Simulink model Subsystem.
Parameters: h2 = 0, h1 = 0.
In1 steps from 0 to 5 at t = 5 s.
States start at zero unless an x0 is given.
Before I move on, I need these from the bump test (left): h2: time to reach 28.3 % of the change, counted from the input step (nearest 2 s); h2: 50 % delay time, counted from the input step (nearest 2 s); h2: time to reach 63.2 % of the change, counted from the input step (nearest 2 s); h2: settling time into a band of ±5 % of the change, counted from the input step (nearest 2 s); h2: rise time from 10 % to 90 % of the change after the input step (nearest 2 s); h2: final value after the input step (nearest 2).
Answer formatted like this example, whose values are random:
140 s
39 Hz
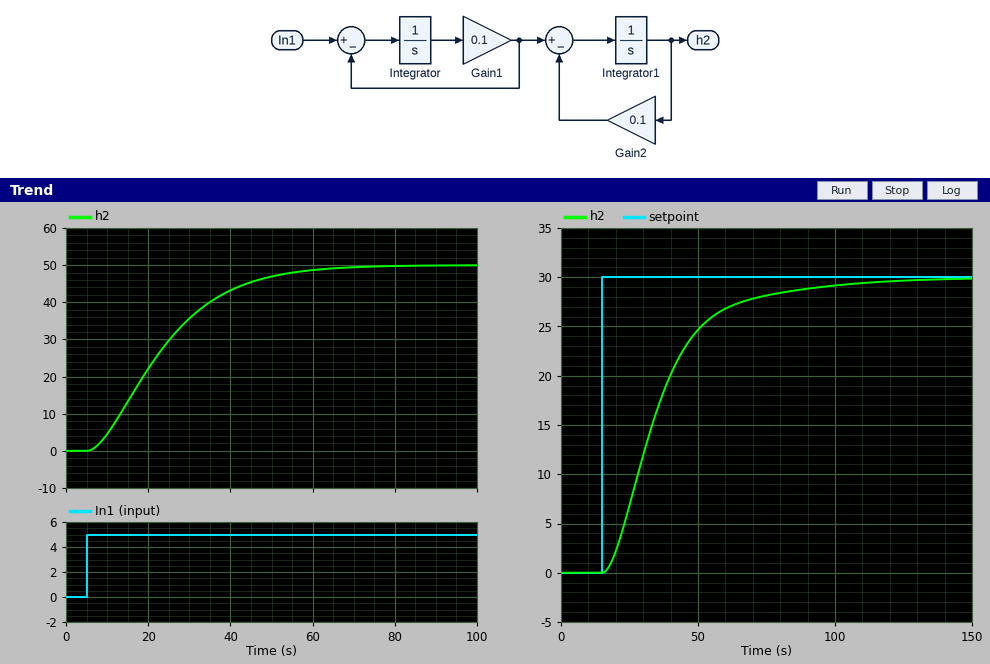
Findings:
10 s
16 s
22 s
48 s
34 s
50
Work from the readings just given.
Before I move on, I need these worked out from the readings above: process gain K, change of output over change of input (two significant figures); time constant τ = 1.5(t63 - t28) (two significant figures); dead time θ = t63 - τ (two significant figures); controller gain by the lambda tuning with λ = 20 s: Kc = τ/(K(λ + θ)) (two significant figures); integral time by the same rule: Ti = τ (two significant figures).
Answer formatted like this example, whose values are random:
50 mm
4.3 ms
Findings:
10
18 s
4.0 s
0.075
18 s
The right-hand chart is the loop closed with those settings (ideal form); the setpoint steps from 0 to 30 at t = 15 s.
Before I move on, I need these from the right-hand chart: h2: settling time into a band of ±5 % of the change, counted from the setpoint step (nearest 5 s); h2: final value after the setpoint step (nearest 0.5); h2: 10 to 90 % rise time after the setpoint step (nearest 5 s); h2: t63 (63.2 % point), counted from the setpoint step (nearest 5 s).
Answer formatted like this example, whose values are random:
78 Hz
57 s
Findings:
65 s
30.0
40 s
25 s
